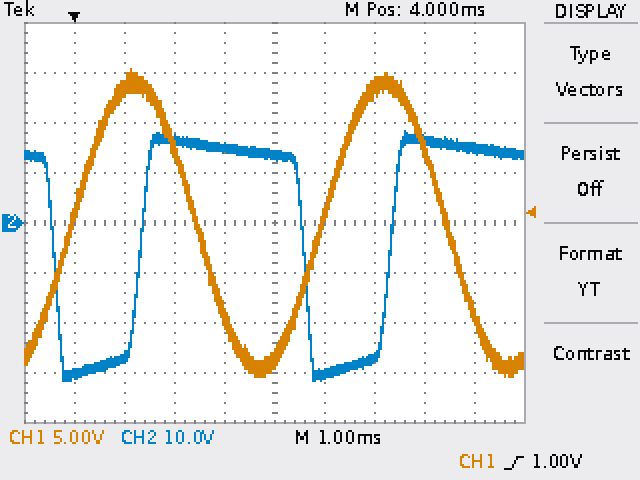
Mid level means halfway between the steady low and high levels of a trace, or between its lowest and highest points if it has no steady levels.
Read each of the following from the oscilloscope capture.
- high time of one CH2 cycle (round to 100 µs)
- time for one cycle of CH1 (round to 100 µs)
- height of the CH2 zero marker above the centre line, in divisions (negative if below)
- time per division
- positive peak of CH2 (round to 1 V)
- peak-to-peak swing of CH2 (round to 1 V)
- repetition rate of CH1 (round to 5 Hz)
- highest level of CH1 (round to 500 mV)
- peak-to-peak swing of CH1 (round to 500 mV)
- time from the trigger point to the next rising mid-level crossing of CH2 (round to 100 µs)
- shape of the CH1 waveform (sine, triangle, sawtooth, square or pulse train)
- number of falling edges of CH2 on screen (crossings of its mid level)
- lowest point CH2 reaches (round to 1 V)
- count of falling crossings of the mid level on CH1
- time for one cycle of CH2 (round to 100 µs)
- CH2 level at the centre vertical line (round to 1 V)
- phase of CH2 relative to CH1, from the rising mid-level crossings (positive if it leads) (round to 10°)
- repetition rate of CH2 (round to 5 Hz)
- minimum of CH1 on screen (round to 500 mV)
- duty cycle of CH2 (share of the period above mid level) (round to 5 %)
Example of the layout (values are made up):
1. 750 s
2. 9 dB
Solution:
1. 3.3 ms
2. 5.0 ms
3. 0.0 div
4. 1 ms
5. 18 V
6. 50 V
7. 200 Hz
8. 15.5 V
9. 31.0 V
10. 1.3 ms
11. sine
12. 2
13. -32 V
14. 2
15. 5.0 ms
16. 13 V
17. -100°
18. 200 Hz
19. -15.5 V
20. 65 %
